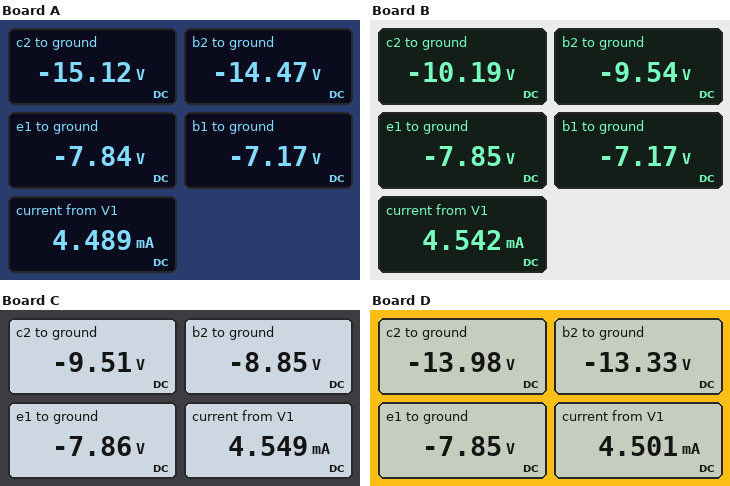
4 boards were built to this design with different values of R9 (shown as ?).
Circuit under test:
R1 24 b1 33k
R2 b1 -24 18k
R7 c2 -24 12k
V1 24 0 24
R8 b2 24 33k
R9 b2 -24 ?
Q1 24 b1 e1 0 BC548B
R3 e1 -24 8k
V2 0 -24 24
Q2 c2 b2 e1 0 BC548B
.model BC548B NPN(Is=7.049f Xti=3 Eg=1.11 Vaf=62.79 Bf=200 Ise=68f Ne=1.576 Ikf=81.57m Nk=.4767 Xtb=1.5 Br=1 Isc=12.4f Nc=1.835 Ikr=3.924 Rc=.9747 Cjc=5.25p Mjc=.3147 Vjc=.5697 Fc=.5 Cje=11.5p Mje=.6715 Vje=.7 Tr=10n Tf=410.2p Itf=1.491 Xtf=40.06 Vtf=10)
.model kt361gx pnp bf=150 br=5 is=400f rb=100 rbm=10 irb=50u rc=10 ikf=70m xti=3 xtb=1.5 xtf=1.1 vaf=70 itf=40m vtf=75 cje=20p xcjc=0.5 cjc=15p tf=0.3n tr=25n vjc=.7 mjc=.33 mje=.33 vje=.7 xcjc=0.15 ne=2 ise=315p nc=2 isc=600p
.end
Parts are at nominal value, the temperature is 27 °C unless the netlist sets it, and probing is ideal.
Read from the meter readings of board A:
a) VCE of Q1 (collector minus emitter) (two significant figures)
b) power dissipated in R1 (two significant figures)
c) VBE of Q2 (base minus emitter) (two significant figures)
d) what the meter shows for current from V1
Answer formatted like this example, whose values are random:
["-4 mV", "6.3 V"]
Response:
["32 V", "29 mW", "-6.6 V", "4.489 mA"]
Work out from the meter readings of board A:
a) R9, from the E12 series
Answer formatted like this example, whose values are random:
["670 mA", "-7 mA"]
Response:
["12 kΩ"]
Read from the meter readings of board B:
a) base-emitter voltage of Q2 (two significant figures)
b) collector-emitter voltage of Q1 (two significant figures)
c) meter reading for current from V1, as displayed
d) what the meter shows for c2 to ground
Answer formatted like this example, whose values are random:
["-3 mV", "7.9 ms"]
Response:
["-1.7 V", "32 V", "4.542 mA", "-10.19 V"]
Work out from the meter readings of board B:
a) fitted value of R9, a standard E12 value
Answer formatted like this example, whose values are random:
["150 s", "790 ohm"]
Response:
["33 kΩ"]
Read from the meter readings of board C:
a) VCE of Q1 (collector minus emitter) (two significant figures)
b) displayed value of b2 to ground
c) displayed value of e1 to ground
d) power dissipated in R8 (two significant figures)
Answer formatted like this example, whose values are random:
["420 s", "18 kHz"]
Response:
["32 V", "-8.85 V", "-7.86 V", "33 mW"]
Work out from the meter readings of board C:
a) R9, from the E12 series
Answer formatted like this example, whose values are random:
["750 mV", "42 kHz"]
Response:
["39 kΩ"]
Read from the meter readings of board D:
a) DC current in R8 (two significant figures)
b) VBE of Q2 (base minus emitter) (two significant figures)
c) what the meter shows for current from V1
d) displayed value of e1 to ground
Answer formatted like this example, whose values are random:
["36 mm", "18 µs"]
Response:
["1.1 mA", "-5.5 V", "4.501 mA", "-7.85 V"]
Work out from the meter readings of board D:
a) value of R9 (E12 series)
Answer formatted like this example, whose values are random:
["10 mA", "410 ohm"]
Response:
["15 kΩ"]
